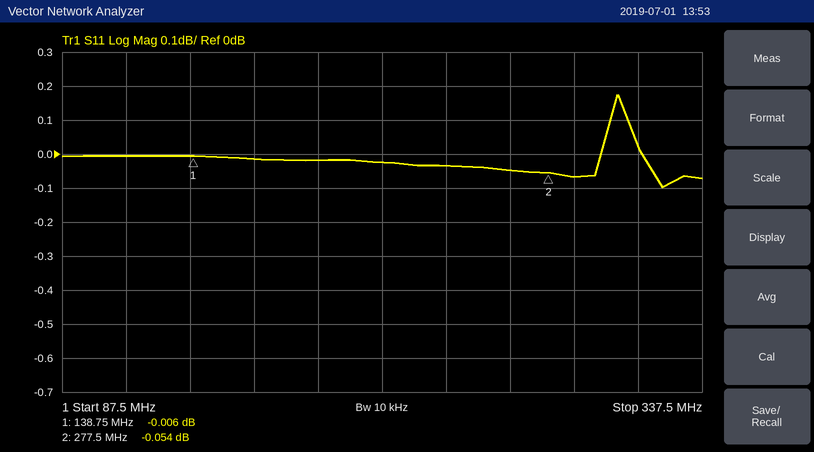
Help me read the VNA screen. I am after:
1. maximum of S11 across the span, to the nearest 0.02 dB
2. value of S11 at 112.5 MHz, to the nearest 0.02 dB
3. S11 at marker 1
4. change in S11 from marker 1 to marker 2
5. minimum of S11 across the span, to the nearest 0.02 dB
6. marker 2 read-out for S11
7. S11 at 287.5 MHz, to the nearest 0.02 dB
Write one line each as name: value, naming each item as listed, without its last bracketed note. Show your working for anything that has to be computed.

maximum of S11 across the span, to the nearest 0.02 dB: 0.18 dB
value of S11 at 112.5 MHz, to the nearest 0.02 dB: 0.00 dB
S11 at marker 1: -0.006 dB
change in S11 from marker 1 to marker 2: -0.054 − (-0.006) = -0.048 dB
minimum of S11 across the span, to the nearest 0.02 dB: -0.10 dB
marker 2 read-out for S11: -0.054 dB
S11 at 287.5 MHz, to the nearest 0.02 dB: -0.06 dB
